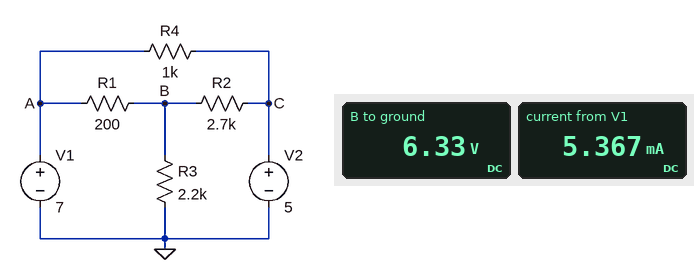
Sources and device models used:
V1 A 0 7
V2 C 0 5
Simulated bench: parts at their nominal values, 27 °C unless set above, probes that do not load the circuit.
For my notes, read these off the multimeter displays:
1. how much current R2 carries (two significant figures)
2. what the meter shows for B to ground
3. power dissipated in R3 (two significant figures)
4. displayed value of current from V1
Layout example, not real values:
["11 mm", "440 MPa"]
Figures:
["490 µA", "6.33 V", "18 mW", "5.367 mA"]
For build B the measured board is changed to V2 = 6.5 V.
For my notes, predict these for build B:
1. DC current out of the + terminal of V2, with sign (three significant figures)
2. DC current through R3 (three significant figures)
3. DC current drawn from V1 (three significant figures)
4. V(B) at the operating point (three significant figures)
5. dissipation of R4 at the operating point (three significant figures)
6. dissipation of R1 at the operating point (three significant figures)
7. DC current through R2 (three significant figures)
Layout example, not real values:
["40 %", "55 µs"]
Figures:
["-471 µA", "2.92 mA", "3.39 mA", "6.42 V", "250 µW", "1.67 mW", "28.9 µA"]
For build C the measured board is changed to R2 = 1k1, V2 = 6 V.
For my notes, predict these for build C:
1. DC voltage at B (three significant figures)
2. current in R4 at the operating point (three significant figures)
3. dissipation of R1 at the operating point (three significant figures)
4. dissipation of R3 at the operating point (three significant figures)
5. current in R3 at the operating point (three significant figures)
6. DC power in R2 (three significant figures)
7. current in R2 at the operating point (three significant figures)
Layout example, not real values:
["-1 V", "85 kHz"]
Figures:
["6.36 V", "1.00 mA", "2.07 mW", "18.4 mW", "2.89 mA", "116 µW", "325 µA"]
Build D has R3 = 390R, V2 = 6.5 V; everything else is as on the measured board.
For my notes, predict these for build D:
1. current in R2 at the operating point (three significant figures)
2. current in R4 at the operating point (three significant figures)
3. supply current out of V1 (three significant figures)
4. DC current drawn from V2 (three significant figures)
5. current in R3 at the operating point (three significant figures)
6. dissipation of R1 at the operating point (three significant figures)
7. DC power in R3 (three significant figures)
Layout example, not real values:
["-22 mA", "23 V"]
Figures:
["661 µA", "500 µA", "11.9 mA", "161 µA", "12.1 mA", "26.1 mW", "57.0 mW"]
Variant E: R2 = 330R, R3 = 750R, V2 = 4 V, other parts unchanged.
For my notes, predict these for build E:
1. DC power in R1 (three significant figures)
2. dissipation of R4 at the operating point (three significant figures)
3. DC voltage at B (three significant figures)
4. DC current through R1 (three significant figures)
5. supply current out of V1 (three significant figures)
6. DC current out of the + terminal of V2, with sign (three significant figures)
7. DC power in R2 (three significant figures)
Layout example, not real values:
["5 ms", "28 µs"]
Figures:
["19.4 mW", "9.00 mW", "5.03 V", "9.84 mA", "12.8 mA", "-6.13 mA", "3.23 mW"]
